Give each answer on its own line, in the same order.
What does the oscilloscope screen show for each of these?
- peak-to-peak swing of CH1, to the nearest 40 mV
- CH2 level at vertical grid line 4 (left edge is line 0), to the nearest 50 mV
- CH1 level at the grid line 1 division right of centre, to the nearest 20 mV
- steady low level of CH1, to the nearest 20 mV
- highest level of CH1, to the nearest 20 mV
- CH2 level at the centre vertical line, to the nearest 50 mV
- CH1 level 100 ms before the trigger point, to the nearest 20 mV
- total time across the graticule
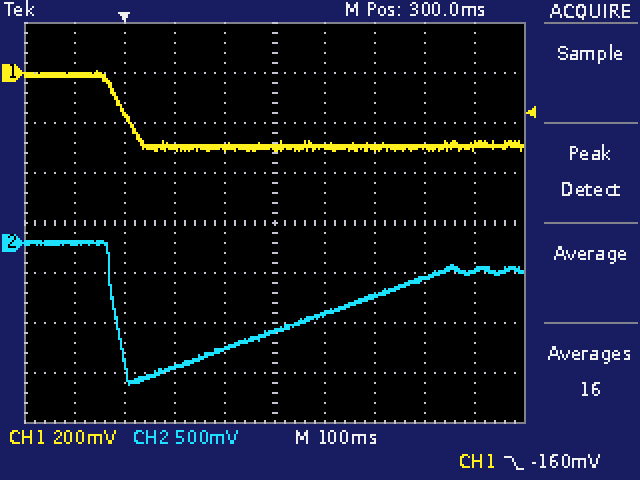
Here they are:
320 mV
-1.05 V
-300 mV
-300 mV
0 mV
-900 mV
0 mV
1 s
